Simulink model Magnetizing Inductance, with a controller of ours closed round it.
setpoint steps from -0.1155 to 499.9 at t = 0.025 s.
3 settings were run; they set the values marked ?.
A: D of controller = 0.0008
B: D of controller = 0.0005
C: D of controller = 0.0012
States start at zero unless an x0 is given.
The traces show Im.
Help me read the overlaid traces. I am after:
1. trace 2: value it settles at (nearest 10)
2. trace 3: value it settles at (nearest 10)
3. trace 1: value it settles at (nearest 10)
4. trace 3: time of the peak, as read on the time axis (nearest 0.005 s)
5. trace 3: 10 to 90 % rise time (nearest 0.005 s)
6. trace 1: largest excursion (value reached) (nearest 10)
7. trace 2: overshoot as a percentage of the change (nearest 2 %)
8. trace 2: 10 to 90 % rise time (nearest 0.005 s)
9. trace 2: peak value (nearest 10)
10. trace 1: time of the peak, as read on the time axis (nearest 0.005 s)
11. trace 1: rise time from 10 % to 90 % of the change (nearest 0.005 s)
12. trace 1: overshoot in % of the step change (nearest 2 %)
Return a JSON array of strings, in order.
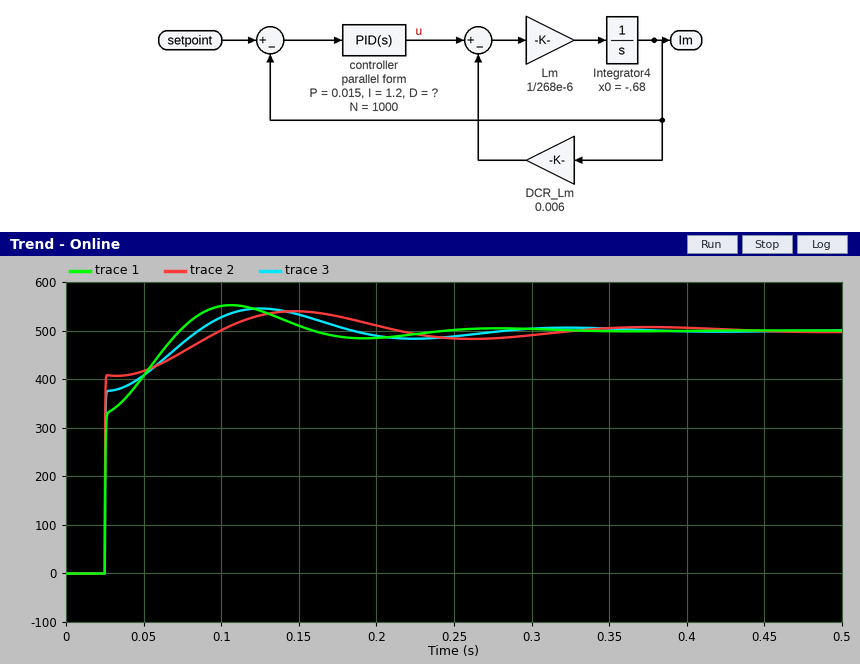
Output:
["500", "500", "500", "0.125 s", "0.040 s", "550", "8 %", "0.045 s", "540", "0.105 s", "0.035 s", "10 %"]
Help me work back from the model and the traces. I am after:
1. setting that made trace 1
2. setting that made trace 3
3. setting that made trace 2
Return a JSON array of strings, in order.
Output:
["B", "A", "C"]
